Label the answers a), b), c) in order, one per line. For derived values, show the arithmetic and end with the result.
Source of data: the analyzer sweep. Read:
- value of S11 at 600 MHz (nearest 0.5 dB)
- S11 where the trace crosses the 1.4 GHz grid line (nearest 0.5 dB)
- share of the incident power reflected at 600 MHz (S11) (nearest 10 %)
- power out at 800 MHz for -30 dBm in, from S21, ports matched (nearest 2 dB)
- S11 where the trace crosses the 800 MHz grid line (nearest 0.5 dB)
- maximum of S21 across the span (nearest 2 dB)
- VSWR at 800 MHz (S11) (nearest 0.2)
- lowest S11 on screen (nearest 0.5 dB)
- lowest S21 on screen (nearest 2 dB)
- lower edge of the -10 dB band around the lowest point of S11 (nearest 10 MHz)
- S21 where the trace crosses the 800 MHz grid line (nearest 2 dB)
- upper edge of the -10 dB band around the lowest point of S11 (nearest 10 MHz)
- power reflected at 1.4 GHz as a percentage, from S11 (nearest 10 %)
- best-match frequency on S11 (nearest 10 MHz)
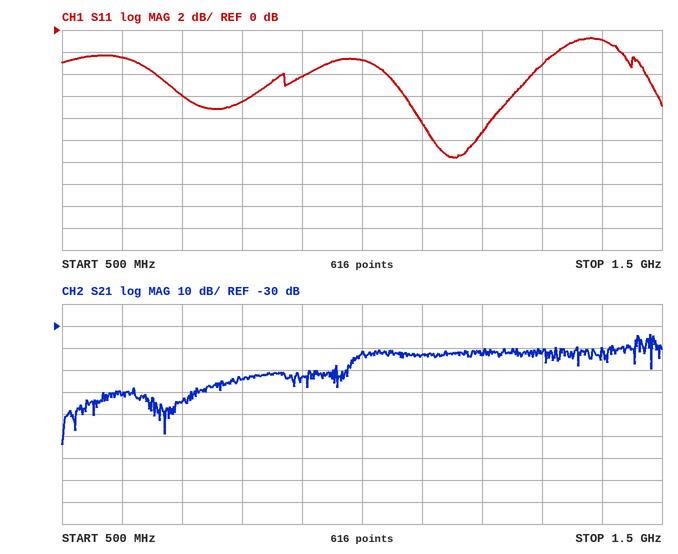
a) -2.5 dB
b) -1.0 dB
c) 10^(-2.5/10) ≈ 56.2 %, so 60 % to the nearest 10 %
d) -30 dBm + (-54 dB) = -84 dBm
e) -6.5 dB
f) -34 dB
g) |Γ| = 10^(-6.5/20) = 0.4732; VSWR = (1 + 0.4732)/(1 − 0.4732) ≈ 2.8
h) -11.5 dB
i) -84 dB
j) 1.12 GHz
k) -54 dB
l) 1.19 GHz
m) 10^(-1/10) ≈ 79.4 %, so 80 % to the nearest 10 %
n) 1.15 GHz
